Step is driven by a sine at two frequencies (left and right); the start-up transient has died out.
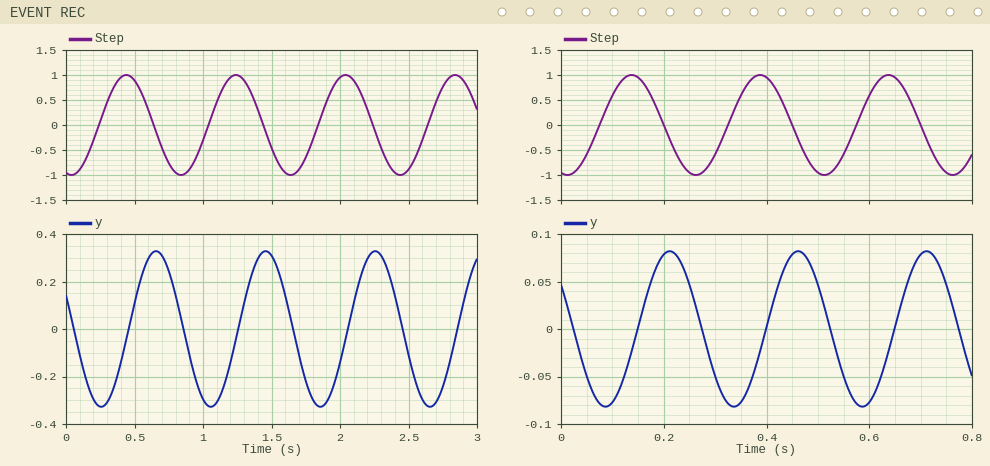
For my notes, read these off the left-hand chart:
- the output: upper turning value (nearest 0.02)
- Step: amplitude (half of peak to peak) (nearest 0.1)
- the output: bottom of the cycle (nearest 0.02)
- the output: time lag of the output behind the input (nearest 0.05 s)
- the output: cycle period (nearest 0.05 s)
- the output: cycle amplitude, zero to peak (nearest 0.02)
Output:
0.32
1.0
-0.32
0.20 s
0.80 s
0.32
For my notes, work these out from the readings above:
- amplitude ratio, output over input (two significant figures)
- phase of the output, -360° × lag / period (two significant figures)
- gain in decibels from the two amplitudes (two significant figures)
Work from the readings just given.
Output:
0.32
-90°
-9.9 dB
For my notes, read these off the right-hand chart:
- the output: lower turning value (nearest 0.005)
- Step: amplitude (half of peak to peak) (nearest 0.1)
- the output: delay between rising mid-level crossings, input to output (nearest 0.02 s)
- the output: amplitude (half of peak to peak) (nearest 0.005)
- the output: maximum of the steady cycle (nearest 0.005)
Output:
-0.080
1.0
0.08 s
0.080
0.080
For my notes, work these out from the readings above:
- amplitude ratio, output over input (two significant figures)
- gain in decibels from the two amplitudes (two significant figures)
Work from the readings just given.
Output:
0.080
-22 dB
